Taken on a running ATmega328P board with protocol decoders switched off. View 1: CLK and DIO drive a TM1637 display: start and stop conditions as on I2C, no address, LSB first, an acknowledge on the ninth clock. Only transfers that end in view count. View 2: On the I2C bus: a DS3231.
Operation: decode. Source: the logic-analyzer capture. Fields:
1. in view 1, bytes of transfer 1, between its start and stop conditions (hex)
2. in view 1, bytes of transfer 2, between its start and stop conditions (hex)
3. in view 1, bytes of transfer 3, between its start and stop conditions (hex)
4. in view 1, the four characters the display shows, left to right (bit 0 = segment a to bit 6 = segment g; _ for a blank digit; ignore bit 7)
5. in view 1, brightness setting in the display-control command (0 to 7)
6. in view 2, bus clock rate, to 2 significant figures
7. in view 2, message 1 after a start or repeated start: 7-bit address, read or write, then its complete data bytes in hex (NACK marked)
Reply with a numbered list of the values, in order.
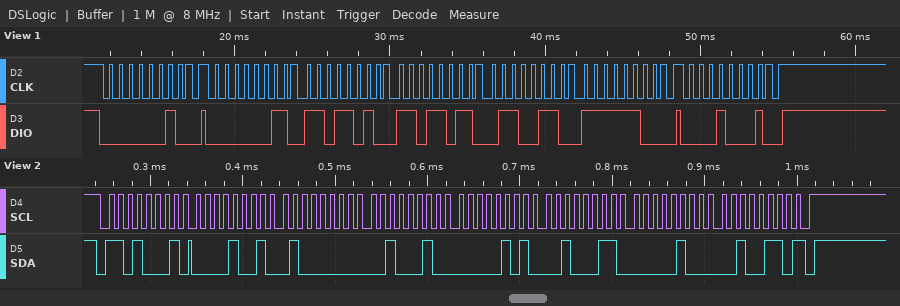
1. 40
2. C0 5B DB 66 3F
3. 88
4. 2240
5. 0
6. 100 kHz
7. 0x68 read: 09 40 22 05 23 04 26 NACK
